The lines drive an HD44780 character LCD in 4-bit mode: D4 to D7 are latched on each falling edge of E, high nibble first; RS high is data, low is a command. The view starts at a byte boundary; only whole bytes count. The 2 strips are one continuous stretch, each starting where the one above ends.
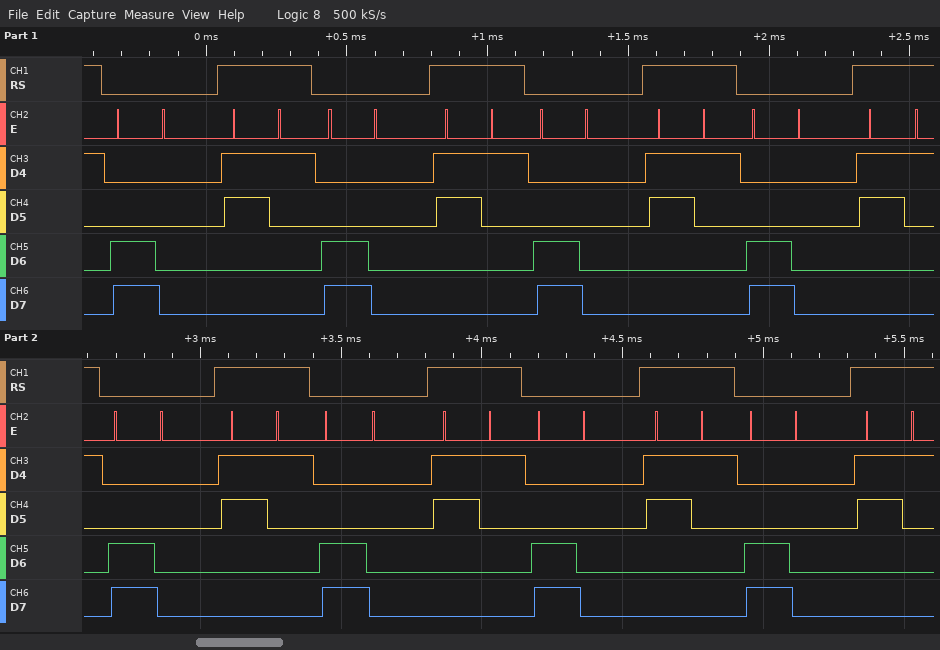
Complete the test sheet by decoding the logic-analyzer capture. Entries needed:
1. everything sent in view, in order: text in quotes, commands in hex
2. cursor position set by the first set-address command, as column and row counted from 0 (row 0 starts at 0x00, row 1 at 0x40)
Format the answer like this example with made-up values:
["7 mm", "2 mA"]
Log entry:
["0xC0 \"1\" 0xC0 \"1\" 0xC0 \"1\" 0xC0 \"1\" 0xC0 \"1\" 0xC0 \"1\" 0xC0 \"1\" 0xC0 \"1\"", "column 0, row 1"]
